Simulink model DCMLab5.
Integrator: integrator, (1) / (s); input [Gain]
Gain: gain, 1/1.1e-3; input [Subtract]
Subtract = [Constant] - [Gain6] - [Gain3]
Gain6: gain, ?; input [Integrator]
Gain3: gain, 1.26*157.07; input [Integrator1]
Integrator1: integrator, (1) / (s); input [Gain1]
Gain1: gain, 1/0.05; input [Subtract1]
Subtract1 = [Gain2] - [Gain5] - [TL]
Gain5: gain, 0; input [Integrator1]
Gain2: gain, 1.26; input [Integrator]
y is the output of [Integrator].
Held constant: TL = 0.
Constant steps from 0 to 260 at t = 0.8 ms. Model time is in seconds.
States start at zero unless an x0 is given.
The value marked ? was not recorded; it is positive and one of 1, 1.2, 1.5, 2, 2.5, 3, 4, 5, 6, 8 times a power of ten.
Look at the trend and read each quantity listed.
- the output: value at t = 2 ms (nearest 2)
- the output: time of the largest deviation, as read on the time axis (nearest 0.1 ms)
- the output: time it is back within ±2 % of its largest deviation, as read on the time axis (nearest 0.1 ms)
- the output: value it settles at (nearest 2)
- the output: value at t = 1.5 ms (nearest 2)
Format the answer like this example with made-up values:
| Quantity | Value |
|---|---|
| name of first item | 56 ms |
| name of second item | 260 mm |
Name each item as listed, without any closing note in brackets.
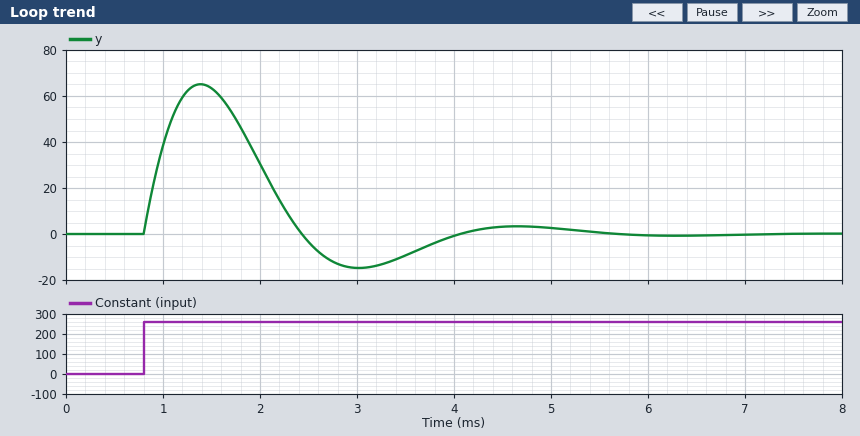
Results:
| Quantity | Value |
|---|---|
| the output: value at t = 2 ms | 30 |
| the output: time of the largest deviation, as read on the time axis | 1.4 ms |
| the output: time it is back within ±2 % of its largest deviation, as read on the time axis | 5.3 ms |
| the output: value it settles at | 0 |
| the output: value at t = 1.5 ms | 64 |
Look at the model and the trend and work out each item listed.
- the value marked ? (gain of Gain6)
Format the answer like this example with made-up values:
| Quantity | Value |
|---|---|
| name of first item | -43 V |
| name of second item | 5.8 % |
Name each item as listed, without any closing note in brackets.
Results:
| Quantity | Value |
|---|---|
| the value marked ? | 2 |
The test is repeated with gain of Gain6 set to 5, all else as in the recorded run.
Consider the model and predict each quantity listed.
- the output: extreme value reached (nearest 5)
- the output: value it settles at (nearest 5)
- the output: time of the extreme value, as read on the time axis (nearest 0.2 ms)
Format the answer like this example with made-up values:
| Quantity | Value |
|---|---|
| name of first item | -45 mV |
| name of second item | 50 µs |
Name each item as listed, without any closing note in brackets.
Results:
| Quantity | Value |
|---|---|
| the output: extreme value reached | 40 |
| the output: value it settles at | 0 |
| the output: time of the extreme value, as read on the time axis | 1.2 ms |
